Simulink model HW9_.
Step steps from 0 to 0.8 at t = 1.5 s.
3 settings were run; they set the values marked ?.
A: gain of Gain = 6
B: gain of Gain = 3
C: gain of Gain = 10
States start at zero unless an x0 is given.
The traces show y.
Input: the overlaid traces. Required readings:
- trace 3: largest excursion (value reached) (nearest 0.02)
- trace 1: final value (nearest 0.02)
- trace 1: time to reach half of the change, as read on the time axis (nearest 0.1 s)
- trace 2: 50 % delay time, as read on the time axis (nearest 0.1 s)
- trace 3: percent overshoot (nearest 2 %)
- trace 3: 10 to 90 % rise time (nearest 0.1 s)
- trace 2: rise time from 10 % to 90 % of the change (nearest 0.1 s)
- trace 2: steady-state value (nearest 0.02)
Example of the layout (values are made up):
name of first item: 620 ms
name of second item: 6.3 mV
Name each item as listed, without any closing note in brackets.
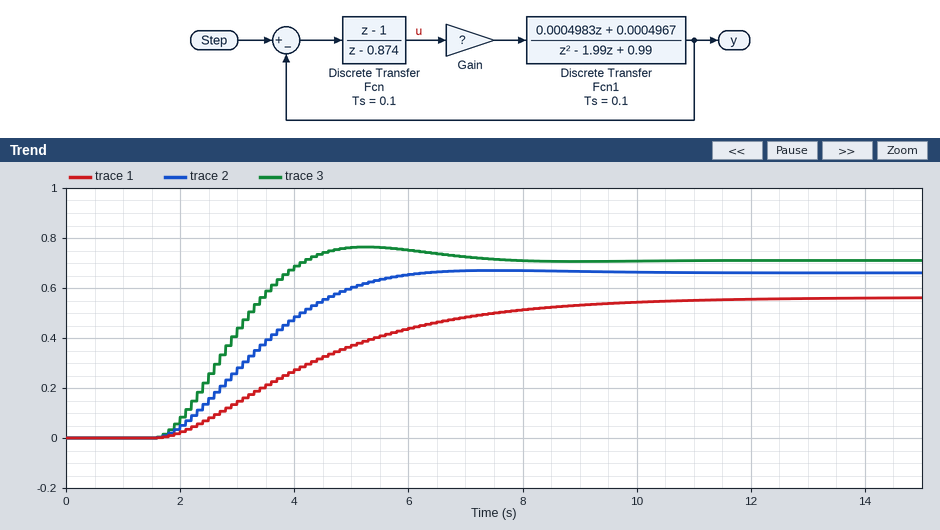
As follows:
trace 3: largest excursion (value reached): 0.76
trace 1: final value: 0.56
trace 1: time to reach half of the change, as read on the time axis: 4.1 s
trace 2: 50 % delay time, as read on the time axis: 3.3 s
trace 3: percent overshoot: 8 %
trace 3: 10 to 90 % rise time: 1.8 s
trace 2: rise time from 10 % to 90 % of the change: 2.8 s
trace 2: steady-state value: 0.66
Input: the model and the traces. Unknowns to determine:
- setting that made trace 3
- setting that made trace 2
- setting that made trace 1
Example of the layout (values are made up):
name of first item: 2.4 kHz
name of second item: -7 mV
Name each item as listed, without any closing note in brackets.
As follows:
setting that made trace 3: C
setting that made trace 2: A
setting that made trace 1: B
